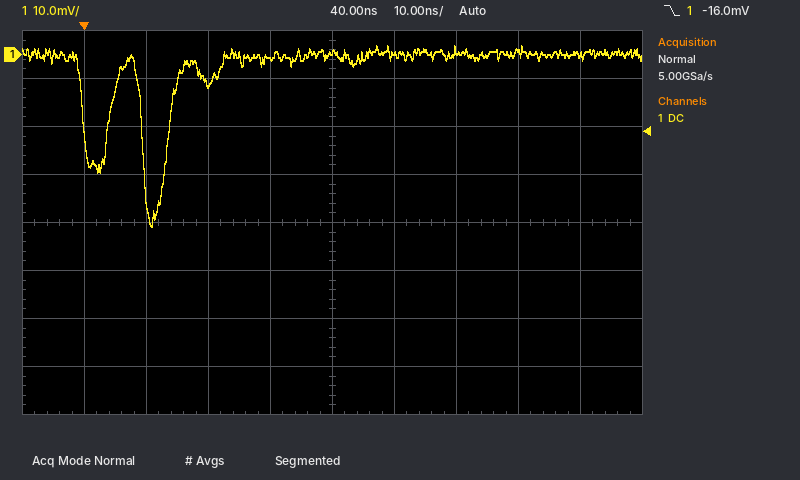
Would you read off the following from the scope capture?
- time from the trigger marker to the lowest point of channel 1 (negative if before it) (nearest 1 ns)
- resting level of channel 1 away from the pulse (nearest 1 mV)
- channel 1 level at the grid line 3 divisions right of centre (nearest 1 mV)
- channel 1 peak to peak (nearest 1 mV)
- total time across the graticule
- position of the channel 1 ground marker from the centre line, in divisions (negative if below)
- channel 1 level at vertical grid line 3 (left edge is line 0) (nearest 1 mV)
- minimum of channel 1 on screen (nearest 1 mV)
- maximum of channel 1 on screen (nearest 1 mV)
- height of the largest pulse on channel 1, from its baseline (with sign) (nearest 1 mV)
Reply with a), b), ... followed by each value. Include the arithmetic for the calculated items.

a) +11 ns
b) 0 mV
c) 0 mV
d) 2 mV − (-36 mV) = 38 mV
e) 100 ns
f) +3.5 div
g) -6 mV
h) -36 mV
i) 2 mV
j) -36 mV − (0 mV) = -36 mV
